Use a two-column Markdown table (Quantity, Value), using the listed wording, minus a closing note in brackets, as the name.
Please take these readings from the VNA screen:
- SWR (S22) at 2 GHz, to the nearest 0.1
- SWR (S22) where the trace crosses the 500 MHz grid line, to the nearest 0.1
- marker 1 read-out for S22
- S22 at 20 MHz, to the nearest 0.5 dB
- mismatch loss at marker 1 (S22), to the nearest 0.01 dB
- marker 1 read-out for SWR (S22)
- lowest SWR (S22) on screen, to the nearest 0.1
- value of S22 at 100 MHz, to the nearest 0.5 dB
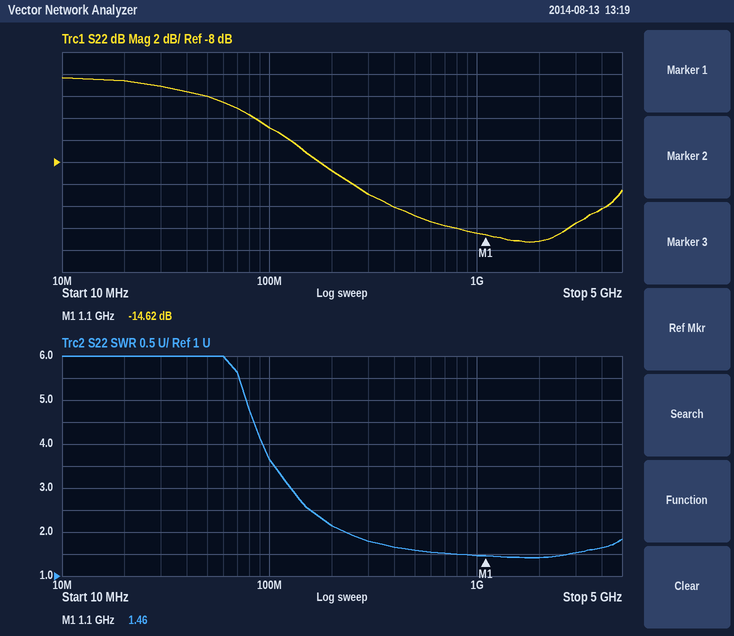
| Quantity | Value |
|---|---|
| SWR (S22) at 2 GHz, to the nearest 0.1 | 1.4 |
| SWR (S22) where the trace crosses the 500 MHz grid line, to the nearest 0.1 | 1.6 |
| marker 1 read-out for S22 | -14.62 dB |
| S22 at 20 MHz, to the nearest 0.5 dB | -0.5 dB |
| mismatch loss at marker 1 (S22), to the nearest 0.01 dB | 0.15 dB |
| marker 1 read-out for SWR | 1.46 |
| lowest SWR (S22) on screen, to the nearest 0.1 | 1.4 |
| value of S22 at 100 MHz, to the nearest 0.5 dB | -5.0 dB |
